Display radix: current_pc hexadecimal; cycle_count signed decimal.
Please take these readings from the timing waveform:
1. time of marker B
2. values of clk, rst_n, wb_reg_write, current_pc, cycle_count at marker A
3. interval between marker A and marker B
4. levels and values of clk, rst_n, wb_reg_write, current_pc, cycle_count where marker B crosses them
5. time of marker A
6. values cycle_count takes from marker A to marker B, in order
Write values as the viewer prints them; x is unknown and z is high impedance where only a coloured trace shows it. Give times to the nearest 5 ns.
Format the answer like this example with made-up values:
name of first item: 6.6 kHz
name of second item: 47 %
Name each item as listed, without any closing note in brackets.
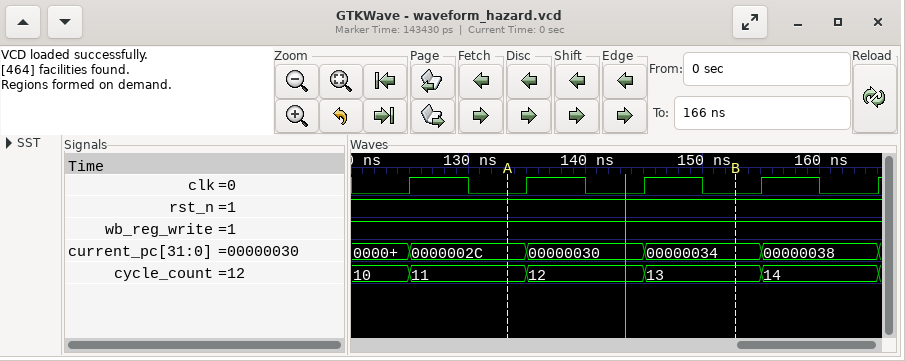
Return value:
time of marker B: 155 ns
values of clk, rst_n, wb_reg_write, current_pc, cycle_count at marker A: clk=0, rst_n=1, wb_reg_write=1, current_pc=0000002C, cycle_count=11
interval between marker A and marker B: 20 ns
levels and values of clk, rst_n, wb_reg_write, current_pc, cycle_count where marker B crosses them: clk=0, rst_n=1, wb_reg_write=1, current_pc=00000034, cycle_count=13
time of marker A: 135 ns
values cycle_count takes from marker A to marker B, in order: 11, 12, 13
